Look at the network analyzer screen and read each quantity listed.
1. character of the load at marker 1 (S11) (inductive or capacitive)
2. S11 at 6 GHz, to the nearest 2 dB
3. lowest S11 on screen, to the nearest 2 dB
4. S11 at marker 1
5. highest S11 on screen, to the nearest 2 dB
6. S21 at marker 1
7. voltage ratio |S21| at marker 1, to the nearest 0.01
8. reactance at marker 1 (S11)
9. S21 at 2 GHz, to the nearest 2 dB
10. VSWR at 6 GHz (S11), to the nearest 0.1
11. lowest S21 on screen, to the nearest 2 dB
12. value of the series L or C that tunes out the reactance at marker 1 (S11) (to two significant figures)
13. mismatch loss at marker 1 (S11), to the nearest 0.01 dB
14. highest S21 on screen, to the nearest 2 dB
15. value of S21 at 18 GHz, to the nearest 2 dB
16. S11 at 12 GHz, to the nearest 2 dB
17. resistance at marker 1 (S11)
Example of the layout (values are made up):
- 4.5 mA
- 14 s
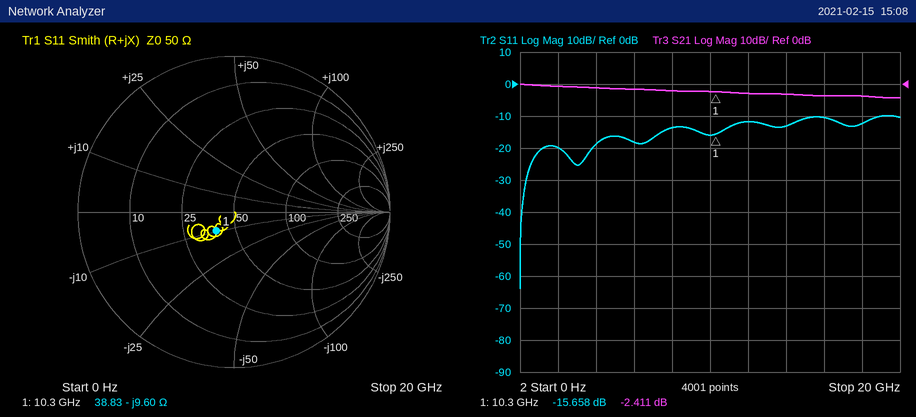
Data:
- capacitive
- -18 dB
- -64 dB
- -15.658 dB
- -10 dB
- -2.411 dB
- 0.76
- -9.60 Ω
- 0 dB
- 1.3
- -4 dB
- 150 pH
- 0.12 dB
- 0 dB
- -4 dB
- -12 dB
- 38.83 Ω
